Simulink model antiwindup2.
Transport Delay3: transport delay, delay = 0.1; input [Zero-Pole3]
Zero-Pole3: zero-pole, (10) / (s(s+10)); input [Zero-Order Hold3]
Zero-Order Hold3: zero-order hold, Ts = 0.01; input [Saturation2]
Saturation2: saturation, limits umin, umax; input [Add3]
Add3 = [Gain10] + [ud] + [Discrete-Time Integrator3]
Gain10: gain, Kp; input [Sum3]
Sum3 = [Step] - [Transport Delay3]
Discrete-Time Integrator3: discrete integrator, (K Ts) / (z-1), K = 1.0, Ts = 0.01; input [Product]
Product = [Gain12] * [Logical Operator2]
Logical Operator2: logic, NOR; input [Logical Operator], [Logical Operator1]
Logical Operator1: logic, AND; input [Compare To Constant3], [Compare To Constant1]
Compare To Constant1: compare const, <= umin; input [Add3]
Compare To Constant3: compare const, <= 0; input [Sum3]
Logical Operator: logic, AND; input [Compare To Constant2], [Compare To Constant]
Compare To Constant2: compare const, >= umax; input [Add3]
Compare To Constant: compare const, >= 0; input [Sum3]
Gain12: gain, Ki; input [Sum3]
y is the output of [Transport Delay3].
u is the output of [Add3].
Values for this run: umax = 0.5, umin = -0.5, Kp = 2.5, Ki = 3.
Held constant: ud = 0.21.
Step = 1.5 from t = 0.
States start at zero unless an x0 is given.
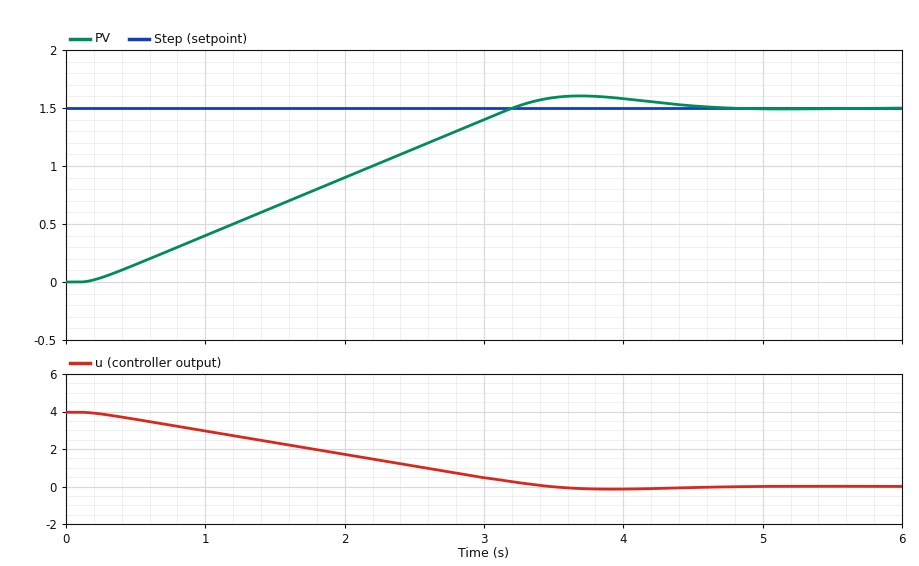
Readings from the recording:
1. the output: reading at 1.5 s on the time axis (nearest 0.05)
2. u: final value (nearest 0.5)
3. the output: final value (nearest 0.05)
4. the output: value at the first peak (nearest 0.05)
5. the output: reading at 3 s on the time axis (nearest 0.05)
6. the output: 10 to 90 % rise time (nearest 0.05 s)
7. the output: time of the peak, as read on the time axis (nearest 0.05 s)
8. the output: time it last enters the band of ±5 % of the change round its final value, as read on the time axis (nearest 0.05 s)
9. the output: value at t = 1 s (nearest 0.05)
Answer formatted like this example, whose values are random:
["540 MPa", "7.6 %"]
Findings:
["0.65", "0.0", "1.50", "1.60", "1.40", "2.40 s", "3.70 s", "4.05 s", "0.40"]
